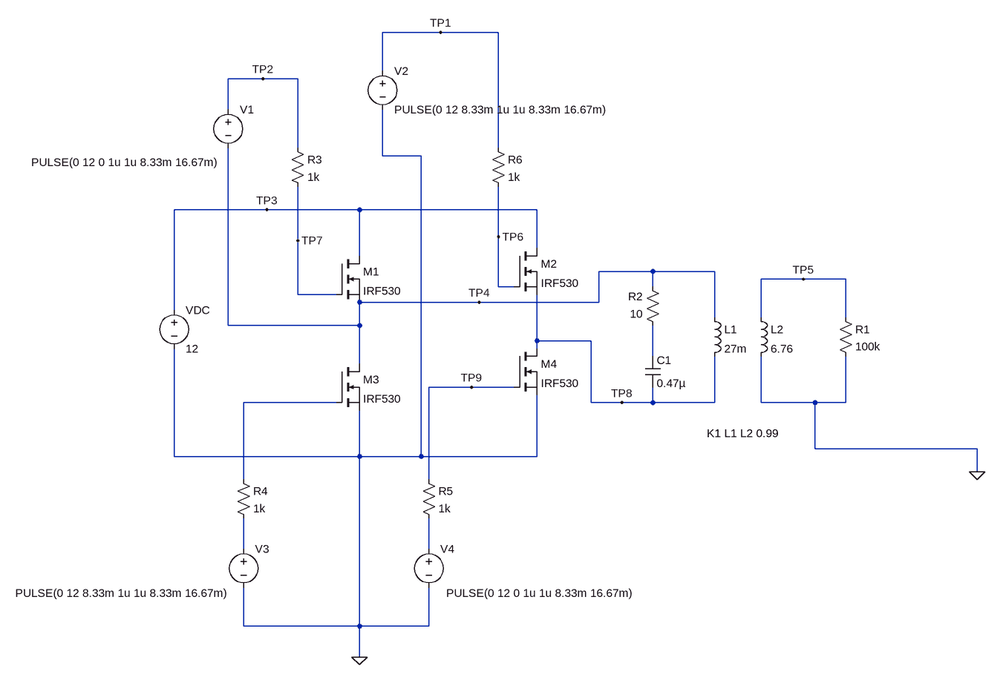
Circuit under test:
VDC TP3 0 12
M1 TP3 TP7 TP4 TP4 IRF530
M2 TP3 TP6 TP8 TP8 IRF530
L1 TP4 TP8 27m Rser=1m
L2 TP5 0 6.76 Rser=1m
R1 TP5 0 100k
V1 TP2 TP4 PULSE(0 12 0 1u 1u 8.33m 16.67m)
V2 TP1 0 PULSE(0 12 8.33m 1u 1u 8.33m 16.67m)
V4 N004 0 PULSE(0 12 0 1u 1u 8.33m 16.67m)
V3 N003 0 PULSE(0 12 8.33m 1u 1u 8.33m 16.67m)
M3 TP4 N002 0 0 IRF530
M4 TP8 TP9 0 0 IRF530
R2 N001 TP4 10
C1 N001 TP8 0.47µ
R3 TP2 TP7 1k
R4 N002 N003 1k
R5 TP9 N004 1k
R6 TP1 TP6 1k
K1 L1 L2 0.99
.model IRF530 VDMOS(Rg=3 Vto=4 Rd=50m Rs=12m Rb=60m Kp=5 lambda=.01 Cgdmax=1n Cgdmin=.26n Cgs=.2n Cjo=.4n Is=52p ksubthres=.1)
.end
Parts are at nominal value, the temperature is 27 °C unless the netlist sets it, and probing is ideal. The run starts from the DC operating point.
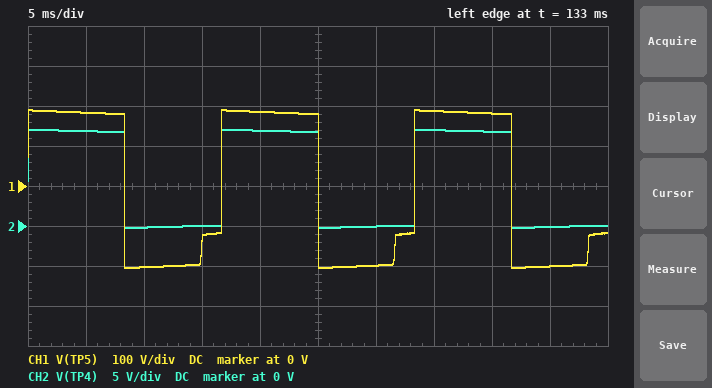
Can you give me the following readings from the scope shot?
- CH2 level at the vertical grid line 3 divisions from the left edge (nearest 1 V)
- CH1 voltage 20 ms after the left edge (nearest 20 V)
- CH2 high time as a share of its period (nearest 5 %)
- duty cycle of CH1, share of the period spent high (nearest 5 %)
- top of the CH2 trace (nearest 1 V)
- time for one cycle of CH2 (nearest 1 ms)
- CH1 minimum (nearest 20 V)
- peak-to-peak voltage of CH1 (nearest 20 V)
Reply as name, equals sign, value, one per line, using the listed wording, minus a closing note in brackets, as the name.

CH2 level at the vertical grid line 3 divisions from the left edge = 0 V
CH1 voltage 20 ms after the left edge = 180 V
CH2 high time as a share of its period = 50 %
duty cycle of CH1, share of the period spent high = 50 %
top of the CH2 trace = 12 V
time for one cycle of CH2 = 17 ms
CH1 minimum = -200 V
peak-to-peak voltage of CH1 = 400 V
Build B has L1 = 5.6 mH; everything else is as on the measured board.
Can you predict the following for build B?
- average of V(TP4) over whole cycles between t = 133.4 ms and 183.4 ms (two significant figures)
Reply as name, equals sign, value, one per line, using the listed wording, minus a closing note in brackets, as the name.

average of V(TP4) over whole cycles between t = 133.4 ms and 183.4 ms = 5.7 V
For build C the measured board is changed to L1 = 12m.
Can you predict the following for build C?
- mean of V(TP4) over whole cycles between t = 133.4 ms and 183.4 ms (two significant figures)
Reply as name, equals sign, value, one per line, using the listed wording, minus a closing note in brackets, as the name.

mean of V(TP4) over whole cycles between t = 133.4 ms and 183.4 ms = 5.8 V
